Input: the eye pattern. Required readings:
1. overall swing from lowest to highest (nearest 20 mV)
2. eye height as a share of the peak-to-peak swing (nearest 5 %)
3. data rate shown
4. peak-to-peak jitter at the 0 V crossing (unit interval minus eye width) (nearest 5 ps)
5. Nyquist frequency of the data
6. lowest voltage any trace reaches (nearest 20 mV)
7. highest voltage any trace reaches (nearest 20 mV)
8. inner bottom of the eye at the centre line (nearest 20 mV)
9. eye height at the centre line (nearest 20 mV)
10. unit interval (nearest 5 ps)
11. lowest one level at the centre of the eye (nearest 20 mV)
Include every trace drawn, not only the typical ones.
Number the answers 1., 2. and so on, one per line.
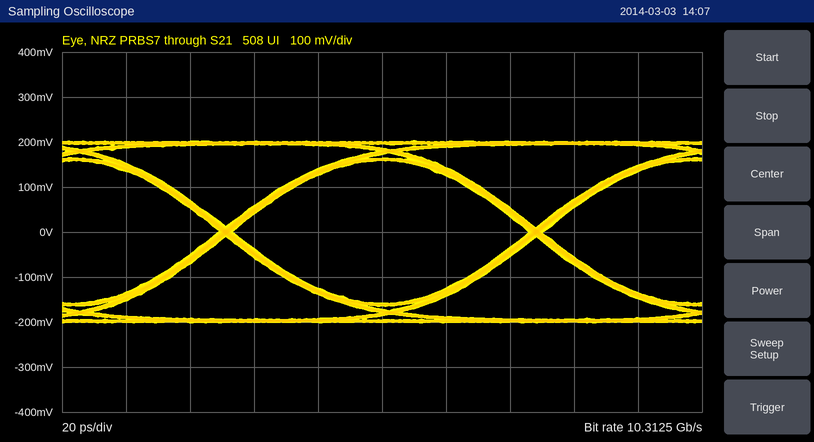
1. 400 mV
2. 80 %
3. 10.3125 Gb/s
4. 5 ps
5. 5.15625 GHz
6. -200 mV
7. 200 mV
8. -160 mV
9. 320 mV
10. 95 ps
11. 160 mV
